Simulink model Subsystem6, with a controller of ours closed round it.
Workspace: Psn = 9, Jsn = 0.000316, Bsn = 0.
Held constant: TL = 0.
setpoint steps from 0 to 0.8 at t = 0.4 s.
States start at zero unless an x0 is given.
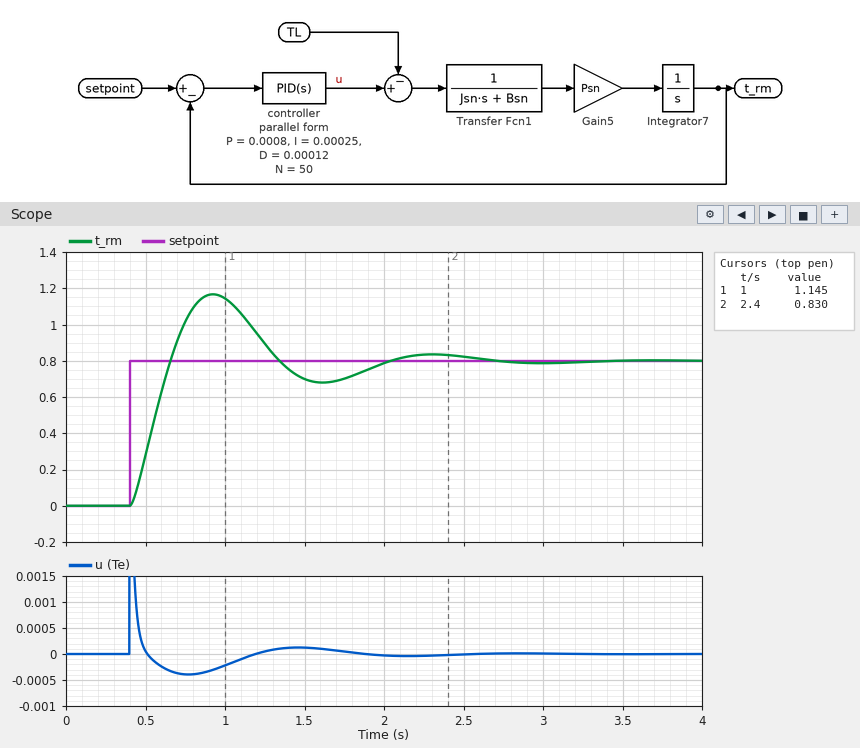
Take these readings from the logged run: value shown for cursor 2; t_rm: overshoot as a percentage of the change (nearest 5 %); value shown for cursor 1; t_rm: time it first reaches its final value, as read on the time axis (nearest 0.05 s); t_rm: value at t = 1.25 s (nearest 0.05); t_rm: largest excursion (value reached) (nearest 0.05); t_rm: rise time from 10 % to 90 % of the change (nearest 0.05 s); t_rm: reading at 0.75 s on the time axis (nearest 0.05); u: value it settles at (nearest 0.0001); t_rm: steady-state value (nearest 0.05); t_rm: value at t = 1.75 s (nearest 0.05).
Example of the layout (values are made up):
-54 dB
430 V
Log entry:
0.830
45 %
1.145
0.65 s
0.90
1.15
0.20 s
1.00
0.0000
0.80
0.70
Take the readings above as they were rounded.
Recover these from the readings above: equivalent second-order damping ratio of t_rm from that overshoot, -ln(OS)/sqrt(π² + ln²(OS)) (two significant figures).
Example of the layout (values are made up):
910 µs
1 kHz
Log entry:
0.25
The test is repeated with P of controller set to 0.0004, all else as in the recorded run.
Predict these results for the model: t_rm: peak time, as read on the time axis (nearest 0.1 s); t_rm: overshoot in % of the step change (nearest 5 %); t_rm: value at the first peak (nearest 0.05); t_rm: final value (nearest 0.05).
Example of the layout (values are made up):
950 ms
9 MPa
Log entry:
1.1 s
40 %
1.10
0.80
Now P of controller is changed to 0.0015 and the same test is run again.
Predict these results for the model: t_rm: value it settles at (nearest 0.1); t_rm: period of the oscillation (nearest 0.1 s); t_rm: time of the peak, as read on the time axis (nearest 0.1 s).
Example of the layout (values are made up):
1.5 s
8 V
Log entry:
0.8
1.0 s
0.8 s
